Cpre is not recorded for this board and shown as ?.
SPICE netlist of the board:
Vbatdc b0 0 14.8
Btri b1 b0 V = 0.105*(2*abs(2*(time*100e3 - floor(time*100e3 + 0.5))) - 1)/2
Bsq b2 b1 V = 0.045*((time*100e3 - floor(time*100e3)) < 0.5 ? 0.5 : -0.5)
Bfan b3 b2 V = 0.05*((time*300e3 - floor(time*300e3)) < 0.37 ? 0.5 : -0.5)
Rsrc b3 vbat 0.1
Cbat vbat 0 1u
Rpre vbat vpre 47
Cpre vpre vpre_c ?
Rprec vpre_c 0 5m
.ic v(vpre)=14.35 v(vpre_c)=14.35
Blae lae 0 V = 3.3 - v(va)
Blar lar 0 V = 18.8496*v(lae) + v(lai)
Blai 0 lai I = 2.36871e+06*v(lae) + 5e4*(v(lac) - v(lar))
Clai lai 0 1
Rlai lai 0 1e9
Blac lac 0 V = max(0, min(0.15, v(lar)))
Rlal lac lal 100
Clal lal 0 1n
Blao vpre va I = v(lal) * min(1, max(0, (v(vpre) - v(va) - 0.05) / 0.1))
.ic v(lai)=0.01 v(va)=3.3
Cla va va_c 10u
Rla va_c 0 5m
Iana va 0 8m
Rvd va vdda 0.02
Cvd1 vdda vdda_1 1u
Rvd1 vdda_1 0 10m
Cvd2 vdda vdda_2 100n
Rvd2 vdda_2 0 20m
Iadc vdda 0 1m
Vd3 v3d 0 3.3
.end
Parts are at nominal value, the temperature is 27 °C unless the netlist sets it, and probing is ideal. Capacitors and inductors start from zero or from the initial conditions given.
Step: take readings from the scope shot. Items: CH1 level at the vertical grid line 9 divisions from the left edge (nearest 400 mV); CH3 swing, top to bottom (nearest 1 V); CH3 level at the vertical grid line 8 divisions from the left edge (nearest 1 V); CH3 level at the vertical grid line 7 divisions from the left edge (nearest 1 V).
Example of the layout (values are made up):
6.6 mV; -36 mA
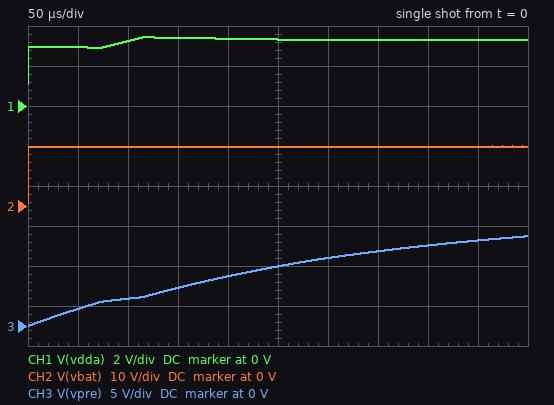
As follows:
3.2 V; 11 V; 10 V; 9 V
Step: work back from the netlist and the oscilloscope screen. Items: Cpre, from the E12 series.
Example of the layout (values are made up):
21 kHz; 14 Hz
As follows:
6.8 µF
